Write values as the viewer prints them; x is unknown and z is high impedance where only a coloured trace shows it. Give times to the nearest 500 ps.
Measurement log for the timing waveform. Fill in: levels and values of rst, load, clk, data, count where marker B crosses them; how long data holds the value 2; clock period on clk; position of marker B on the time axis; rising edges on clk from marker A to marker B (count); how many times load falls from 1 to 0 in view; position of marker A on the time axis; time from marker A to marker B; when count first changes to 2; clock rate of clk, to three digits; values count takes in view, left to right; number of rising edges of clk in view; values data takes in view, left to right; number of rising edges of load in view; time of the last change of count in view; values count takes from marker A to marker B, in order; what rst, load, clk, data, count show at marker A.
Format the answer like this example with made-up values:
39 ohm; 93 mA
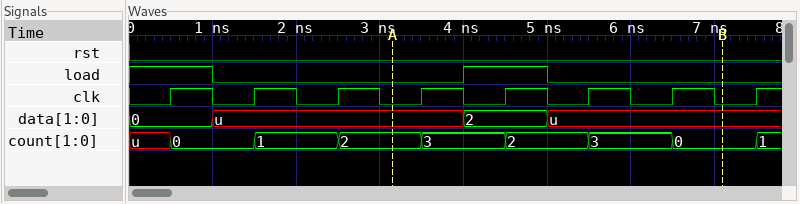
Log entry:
rst=0, load=0, clk=0, data=u, count=0; 1000 ps; 1000 ps; 7000 ps; 4; 2; 3000 ps; 4000 ps; 2500 ps; 1.00 GHz; u, 0, 1, 2, 3, 2, 3, 0, 1; 8; 0, u, 2, u; 1; 7500 ps; 2, 3, 2, 3, 0; rst=0, load=0, clk=0, data=u, count=2
